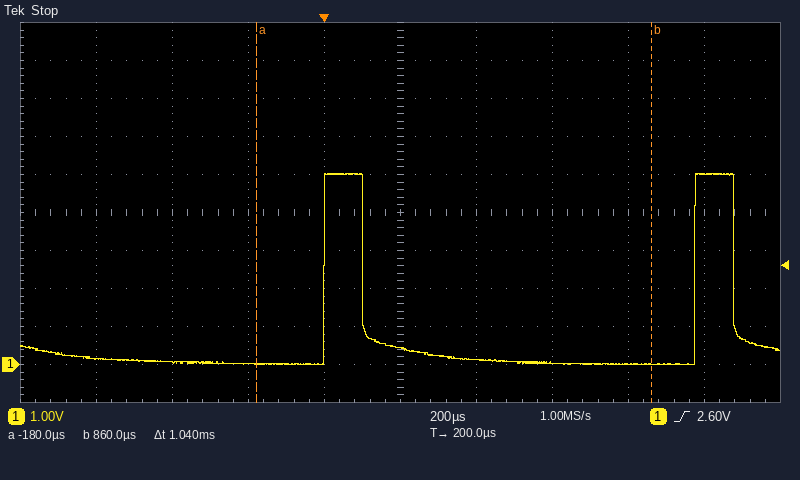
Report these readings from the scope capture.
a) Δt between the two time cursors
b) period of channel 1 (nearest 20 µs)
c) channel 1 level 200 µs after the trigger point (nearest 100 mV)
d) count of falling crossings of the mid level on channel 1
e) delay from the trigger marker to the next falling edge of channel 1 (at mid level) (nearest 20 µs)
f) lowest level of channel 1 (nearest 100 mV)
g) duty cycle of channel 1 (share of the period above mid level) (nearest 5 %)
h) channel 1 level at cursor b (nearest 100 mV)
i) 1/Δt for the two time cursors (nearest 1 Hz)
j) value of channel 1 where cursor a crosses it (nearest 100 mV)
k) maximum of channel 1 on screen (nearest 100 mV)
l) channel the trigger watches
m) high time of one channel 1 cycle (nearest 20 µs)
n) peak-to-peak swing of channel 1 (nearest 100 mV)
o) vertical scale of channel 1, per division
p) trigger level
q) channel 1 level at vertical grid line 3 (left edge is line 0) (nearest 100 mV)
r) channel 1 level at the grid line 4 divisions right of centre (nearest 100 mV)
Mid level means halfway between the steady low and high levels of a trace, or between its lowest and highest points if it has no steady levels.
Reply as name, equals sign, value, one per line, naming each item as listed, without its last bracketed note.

Δt between the two time cursors = 1.04 ms
period of channel 1 = 980 µs
channel 1 level 200 µs after the trigger point = 400 mV
count of falling crossings of the mid level on channel 1 = 2
delay from the trigger marker to the next falling edge of channel 1 (at mid level) = 100 µs
lowest level of channel 1 = 0.0 V
duty cycle of channel 1 (share of the period above mid level) = 10 %
channel 1 level at cursor b = 0.0 V
1/Δt for the two time cursors = 962 Hz
value of channel 1 where cursor a crosses it = 0.0 V
maximum of channel 1 on screen = 5.0 V
channel the trigger watches = channel 1
high time of one channel 1 cycle = 100 µs
peak-to-peak swing of channel 1 = 5.0 V
vertical scale of channel 1, per division = 1 V
trigger level = 2.60 V
channel 1 level at vertical grid line 3 (left edge is line 0) = 0.0 V
channel 1 level at the grid line 4 divisions right of centre = 5.0 V
